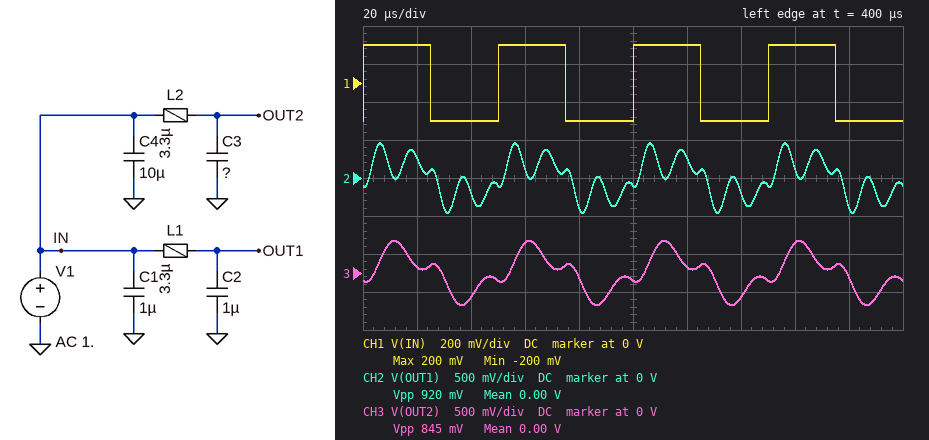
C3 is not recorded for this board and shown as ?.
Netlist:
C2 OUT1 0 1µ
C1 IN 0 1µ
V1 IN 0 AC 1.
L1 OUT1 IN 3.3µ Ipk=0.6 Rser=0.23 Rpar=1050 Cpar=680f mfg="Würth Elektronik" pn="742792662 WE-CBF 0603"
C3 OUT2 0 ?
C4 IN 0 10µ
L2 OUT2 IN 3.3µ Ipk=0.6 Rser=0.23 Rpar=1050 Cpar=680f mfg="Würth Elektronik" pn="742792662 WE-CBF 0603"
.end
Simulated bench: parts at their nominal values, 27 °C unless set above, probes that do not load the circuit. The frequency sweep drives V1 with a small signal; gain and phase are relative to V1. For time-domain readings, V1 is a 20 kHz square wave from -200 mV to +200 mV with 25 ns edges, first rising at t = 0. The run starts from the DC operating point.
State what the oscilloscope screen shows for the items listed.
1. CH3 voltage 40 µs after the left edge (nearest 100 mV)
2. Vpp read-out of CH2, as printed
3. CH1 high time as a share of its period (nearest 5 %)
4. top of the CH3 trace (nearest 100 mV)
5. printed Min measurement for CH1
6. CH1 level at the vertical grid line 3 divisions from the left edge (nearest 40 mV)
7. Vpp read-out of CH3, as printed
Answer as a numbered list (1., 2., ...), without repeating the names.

1. -300 mV
2. 920 mV
3. 50 %
4. 400 mV
5. -200 mV
6. 200 mV
7. 845 mV
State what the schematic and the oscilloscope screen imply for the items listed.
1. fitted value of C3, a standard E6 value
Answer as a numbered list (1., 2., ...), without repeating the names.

1. 3.3 µF
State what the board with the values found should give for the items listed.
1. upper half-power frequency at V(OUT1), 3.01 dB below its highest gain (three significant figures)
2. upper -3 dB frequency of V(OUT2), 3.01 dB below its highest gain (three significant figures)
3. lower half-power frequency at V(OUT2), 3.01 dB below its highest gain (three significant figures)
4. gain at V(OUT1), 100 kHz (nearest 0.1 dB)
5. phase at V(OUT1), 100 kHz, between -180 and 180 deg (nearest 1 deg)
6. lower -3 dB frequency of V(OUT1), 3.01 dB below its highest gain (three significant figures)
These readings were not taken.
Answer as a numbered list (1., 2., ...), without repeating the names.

1. 92.7 kHz
2. 52.9 kHz
3. 41.6 kHz
4. 9.5 dB
5. -154 deg
6. 81.4 kHz
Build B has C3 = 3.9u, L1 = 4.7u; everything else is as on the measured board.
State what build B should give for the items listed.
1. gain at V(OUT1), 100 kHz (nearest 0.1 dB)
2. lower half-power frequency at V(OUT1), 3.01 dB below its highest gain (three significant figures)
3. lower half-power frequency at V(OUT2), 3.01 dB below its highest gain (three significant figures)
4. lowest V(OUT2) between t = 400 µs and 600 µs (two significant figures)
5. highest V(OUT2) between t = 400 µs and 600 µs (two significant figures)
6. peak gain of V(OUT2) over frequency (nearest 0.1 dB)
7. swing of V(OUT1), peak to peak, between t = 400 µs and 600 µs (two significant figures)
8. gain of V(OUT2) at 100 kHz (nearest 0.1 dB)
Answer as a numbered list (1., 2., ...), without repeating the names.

1. 1.2 dB
2. 69.1 kHz
3. 37.6 kHz
4. -390 mV
5. 390 mV
6. 12.1 dB
7. 910 mV
8. -12.3 dB
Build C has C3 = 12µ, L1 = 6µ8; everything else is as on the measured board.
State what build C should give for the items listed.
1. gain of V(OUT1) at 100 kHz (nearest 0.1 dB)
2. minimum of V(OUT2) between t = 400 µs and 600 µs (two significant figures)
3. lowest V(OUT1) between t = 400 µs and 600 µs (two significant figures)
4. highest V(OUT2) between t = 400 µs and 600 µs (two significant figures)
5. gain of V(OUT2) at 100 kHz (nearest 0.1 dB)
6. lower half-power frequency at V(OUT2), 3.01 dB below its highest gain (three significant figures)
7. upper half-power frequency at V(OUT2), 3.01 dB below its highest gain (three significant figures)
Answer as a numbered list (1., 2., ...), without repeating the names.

1. -4.6 dB
2. -490 mV
3. -1.1 V
4. 490 mV
5. -23.4 dB
6. 17.4 kHz
7. 29.2 kHz
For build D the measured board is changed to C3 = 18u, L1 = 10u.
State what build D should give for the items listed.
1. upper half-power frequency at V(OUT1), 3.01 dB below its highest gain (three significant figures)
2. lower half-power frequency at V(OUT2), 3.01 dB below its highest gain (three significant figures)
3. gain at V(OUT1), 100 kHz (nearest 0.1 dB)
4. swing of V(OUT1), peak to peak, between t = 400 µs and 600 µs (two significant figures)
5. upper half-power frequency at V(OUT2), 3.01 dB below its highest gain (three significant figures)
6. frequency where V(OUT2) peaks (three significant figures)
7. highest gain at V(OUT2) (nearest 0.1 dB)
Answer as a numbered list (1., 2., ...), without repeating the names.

1. 52.1 kHz
2. 12.0 kHz
3. -9.4 dB
4. 970 mV
5. 24.2 kHz
6. 19.1 kHz
7. 5.7 dB
